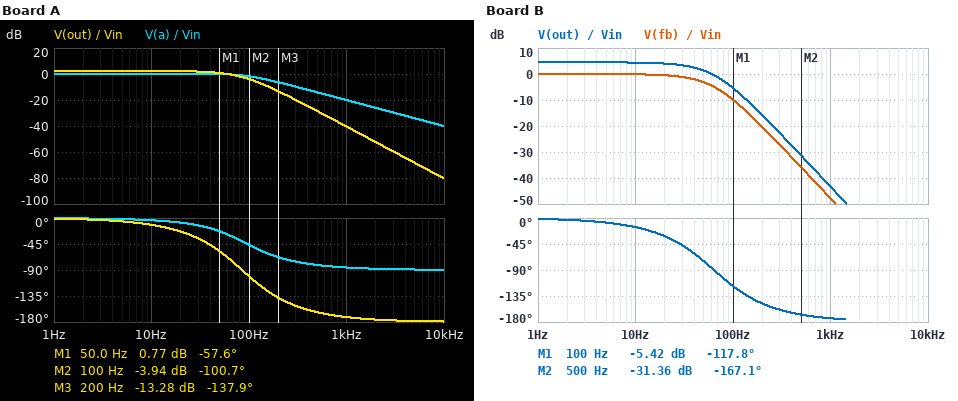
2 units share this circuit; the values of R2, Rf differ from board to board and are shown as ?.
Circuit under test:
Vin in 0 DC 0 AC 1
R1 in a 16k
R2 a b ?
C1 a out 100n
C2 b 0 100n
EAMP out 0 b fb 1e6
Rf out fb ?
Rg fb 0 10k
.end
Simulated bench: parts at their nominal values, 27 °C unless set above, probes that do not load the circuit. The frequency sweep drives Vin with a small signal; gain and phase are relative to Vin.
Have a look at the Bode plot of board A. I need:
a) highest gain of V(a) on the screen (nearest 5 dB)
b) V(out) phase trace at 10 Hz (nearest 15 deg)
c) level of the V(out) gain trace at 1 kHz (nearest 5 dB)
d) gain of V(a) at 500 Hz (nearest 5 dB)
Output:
0 dB
-15 deg
-40 dB
-15 dB
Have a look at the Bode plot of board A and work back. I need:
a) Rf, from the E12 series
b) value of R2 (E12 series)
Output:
3.3 kΩ
22 kΩ
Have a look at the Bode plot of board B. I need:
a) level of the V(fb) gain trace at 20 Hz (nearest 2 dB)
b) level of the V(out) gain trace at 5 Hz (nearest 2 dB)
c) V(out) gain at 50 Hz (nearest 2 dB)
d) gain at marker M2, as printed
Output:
0 dB
4 dB
2 dB
-31.36 dB
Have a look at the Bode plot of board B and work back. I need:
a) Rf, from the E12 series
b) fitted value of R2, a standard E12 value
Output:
6.8 kΩ
39 kΩ
